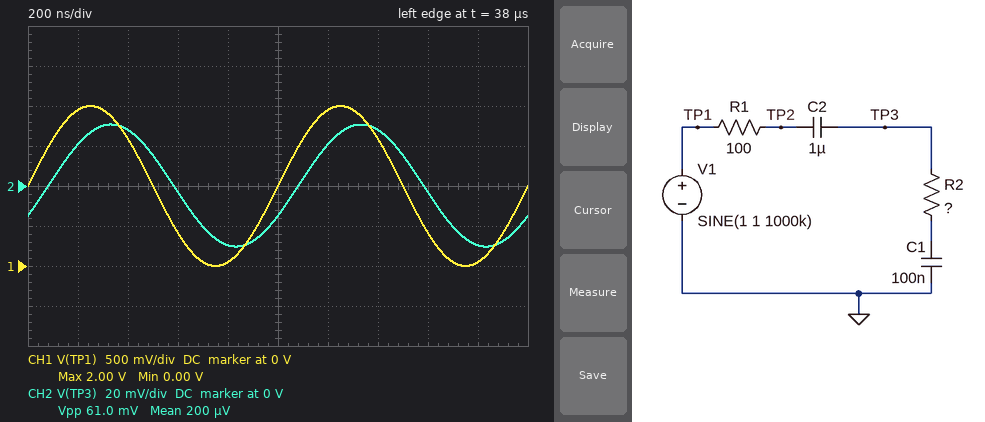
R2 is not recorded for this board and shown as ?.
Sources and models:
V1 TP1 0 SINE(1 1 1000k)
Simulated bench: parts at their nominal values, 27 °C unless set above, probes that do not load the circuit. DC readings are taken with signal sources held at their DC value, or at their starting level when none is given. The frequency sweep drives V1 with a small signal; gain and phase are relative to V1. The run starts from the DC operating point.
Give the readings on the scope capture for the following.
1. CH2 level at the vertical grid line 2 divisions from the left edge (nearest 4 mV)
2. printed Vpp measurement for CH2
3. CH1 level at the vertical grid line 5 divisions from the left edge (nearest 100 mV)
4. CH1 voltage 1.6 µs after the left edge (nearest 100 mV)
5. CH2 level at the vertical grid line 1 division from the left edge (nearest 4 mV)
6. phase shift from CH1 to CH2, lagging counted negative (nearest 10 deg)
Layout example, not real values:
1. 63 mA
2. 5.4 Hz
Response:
1. 28 mV
2. 61.0 mV
3. 1.0 V
4. 400 mV
5. 20 mV
6. -30 deg
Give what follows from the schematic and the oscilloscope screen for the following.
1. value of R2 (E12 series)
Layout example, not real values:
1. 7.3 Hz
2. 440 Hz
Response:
1. 2.7 Ω
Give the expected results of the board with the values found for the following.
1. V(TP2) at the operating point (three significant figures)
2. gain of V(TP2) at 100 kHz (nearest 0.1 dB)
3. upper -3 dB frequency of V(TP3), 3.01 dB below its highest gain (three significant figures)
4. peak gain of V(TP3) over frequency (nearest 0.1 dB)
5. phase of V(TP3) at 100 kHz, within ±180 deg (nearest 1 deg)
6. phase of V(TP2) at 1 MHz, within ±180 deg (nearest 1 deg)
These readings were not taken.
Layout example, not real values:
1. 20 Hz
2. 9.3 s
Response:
1. 1.00 V
2. -15.4 dB
3. 17.1 kHz
4. -0.8 dB
5. -71 deg
6. -32 deg
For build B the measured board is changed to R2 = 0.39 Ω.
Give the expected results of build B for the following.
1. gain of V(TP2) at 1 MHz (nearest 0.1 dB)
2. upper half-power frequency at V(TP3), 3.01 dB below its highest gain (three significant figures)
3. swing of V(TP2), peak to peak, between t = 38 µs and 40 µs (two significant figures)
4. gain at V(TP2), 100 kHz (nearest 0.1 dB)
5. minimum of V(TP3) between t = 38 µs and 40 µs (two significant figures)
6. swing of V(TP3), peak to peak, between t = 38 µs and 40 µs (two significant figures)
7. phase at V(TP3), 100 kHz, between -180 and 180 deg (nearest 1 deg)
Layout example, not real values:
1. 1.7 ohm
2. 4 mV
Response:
1. -35.0 dB
2. 17.4 kHz
3. 36 mV
4. -15.3 dB
5. -16 mV
6. 33 mV
7. -79 deg
